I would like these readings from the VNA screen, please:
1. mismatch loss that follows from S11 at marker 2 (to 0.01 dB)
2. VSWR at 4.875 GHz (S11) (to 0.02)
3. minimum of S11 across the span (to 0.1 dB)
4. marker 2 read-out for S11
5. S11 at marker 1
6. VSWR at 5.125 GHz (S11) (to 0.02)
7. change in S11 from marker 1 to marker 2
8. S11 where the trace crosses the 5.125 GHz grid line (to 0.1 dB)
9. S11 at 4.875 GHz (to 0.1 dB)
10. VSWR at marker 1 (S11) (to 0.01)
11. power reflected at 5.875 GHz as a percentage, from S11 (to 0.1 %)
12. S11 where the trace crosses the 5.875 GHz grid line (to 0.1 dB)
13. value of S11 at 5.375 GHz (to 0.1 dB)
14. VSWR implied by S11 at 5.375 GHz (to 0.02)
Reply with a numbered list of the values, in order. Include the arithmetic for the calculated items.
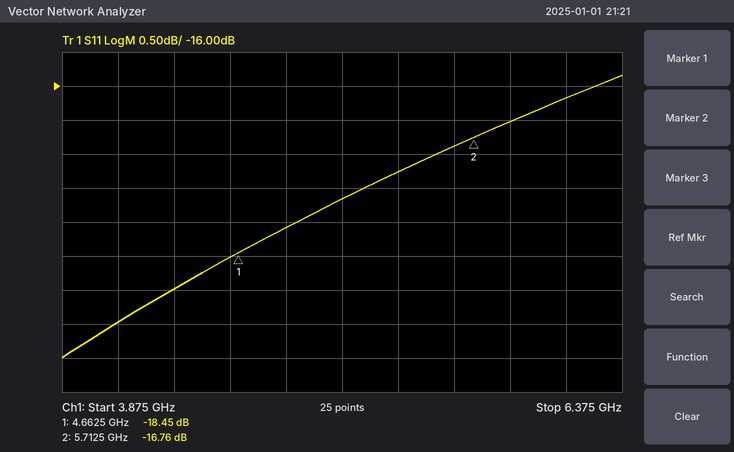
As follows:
1. −10 log10(1 − 10^(-16.76/10)) ≈ 0.09 dB
2. |Γ| = 10^(-18.1/20) = 0.1245; VSWR = (1 + 0.1245)/(1 − 0.1245) ≈ 1.28
3. -20.0 dB
4. -16.76 dB
5. -18.45 dB
6. |Γ| = 10^(-17.7/20) = 0.1303; VSWR = (1 + 0.1303)/(1 − 0.1303) ≈ 1.30
7. -16.76 − (-18.45) = 1.69 dB
8. -17.7 dB
9. -18.1 dB
10. (1 + 0.1195)/(1 − 0.1195) ≈ 1.27
11. 10^(-16.5/10) ≈ 2.2 %
12. -16.5 dB
13. -17.3 dB
14. |Γ| = 10^(-17.3/20) = 0.1365; VSWR = (1 + 0.1365)/(1 − 0.1365) ≈ 1.32
